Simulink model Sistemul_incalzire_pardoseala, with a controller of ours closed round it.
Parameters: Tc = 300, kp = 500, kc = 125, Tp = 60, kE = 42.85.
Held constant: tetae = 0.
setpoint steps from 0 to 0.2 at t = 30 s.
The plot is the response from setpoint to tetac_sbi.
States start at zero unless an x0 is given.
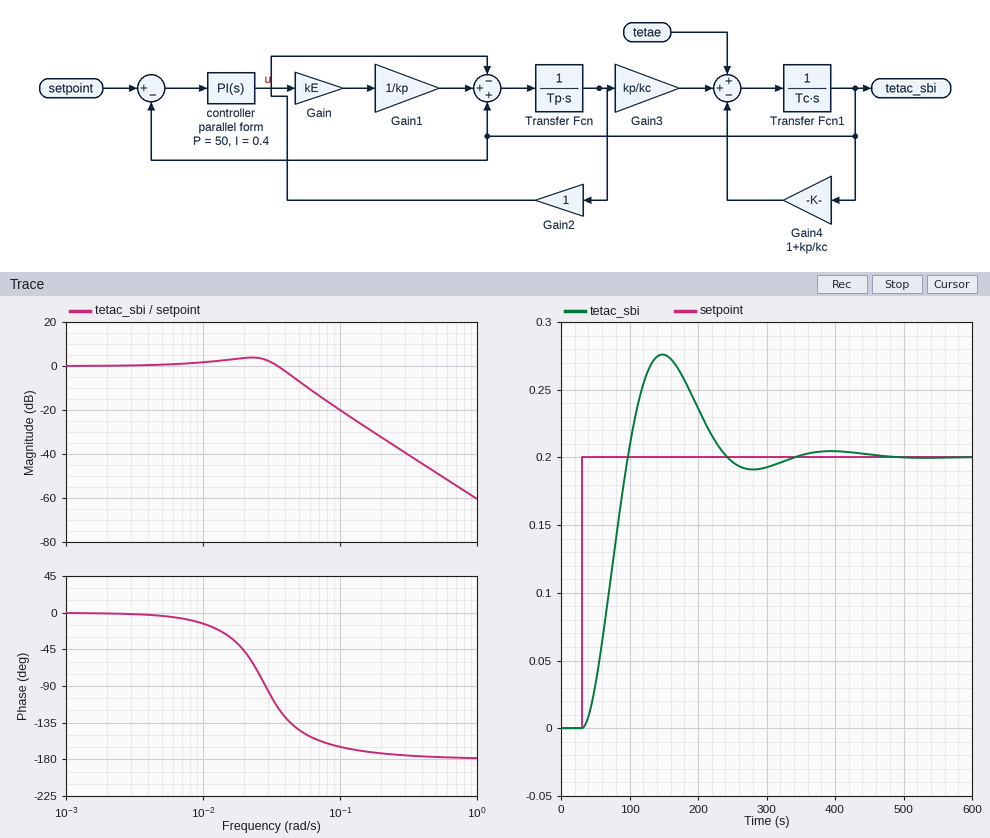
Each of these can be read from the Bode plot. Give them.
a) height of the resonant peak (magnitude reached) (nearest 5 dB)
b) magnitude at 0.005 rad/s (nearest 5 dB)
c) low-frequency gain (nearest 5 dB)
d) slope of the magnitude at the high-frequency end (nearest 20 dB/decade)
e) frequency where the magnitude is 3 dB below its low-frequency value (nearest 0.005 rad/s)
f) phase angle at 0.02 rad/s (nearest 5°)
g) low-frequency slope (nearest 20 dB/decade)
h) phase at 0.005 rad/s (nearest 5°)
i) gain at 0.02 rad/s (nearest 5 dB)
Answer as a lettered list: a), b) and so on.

a) 5 dB
b) 0 dB
c) 0 dB
d) -40 dB/decade
e) 0.040 rad/s
f) -45°
g) 0 dB/decade
h) -5°
i) 5 dB
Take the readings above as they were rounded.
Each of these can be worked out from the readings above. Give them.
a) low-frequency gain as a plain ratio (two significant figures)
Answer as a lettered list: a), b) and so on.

a) 1.0
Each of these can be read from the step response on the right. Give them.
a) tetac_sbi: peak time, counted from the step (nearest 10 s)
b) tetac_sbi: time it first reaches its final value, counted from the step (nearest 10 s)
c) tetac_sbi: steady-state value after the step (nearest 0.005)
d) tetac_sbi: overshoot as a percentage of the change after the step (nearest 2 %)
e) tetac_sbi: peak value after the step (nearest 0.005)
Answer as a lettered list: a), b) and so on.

a) 120 s
b) 70 s
c) 0.200
d) 38 %
e) 0.275
